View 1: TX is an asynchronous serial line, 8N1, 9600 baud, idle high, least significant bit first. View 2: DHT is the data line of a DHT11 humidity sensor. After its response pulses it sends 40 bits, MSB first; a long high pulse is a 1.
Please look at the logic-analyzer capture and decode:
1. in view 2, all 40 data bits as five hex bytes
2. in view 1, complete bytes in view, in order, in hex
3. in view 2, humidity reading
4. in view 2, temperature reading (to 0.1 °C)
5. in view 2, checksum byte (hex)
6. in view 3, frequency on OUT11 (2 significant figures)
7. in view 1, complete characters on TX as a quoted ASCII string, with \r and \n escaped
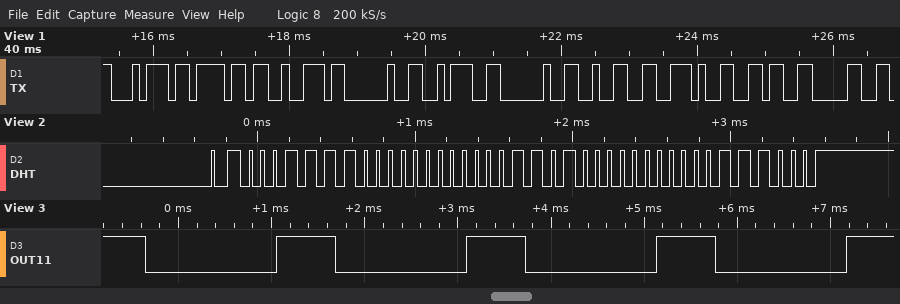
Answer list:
1E 00 1A 00 38
0x74 0x6F 0x72 0x20 0x3A 0x20 0x32 0x2E 0x36 0x30
30 %
26.0 °C
0x38
490 Hz
"tor : 2.60"
